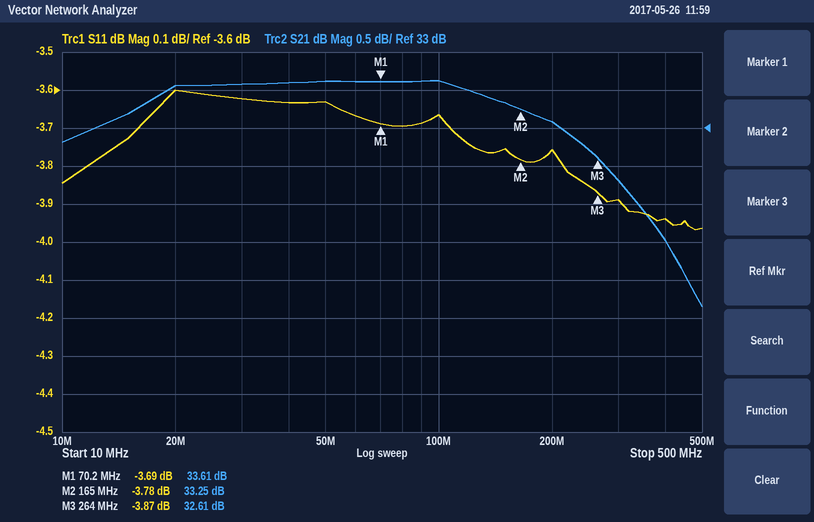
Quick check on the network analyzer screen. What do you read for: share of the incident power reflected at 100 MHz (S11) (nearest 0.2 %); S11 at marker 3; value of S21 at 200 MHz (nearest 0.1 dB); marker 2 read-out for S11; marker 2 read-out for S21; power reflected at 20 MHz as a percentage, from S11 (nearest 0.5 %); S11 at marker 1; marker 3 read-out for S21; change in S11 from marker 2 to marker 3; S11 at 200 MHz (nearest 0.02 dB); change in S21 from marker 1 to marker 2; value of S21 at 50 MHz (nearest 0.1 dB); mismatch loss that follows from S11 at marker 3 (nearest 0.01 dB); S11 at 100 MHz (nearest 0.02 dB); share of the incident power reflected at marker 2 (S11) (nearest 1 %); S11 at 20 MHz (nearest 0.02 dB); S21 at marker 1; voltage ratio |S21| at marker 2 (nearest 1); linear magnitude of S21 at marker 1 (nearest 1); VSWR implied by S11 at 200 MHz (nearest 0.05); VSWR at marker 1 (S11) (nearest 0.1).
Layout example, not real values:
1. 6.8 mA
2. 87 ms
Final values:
1. 43.0 %
2. -3.87 dB
3. 33.1 dB
4. -3.78 dB
5. 33.25 dB
6. 43.5 %
7. -3.69 dB
8. 32.61 dB
9. -0.09 dB
10. -3.76 dB
11. -0.36 dB
12. 33.6 dB
13. 2.29 dB
14. -3.66 dB
15. 42 %
16. -3.60 dB
17. 33.61 dB
18. 46
19. 48
20. 4.70
21. 4.8
